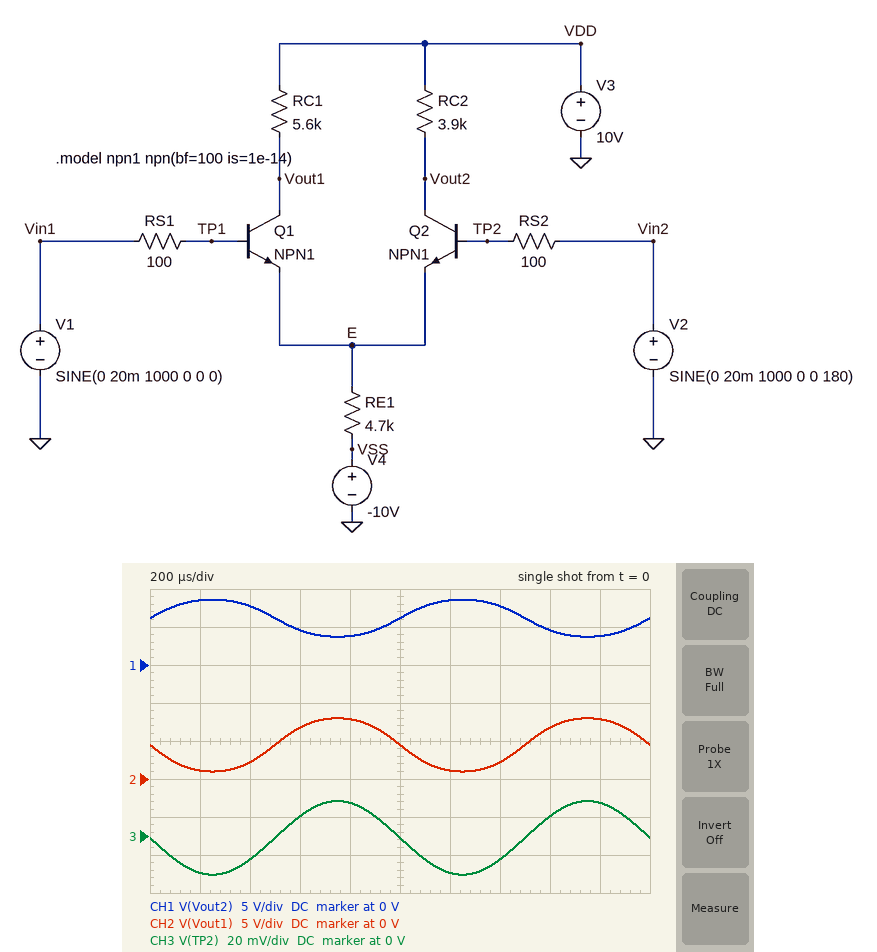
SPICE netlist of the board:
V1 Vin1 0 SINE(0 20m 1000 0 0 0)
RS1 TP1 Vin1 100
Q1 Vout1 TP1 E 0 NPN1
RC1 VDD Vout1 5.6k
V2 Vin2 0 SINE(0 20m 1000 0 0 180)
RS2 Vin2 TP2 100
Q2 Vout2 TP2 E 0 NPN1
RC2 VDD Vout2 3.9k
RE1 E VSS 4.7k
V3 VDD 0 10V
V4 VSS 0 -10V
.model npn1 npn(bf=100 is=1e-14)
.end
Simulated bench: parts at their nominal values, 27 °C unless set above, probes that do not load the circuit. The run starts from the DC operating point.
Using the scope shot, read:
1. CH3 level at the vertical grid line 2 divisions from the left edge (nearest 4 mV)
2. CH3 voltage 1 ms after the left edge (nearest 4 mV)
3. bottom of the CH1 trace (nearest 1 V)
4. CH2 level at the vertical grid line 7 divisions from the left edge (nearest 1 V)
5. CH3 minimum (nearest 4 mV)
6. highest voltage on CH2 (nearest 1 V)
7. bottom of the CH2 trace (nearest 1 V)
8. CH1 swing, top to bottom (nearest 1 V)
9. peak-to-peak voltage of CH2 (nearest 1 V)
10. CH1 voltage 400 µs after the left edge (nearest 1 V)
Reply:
-12 mV
0 V
4 V
2 V
-20 mV
8 V
1 V
5 V
7 V
8 V
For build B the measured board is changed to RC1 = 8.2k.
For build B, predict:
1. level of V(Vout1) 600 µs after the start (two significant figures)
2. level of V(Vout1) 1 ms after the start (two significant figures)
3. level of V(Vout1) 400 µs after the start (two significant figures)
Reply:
5.3 V
1.9 V
-560 mV
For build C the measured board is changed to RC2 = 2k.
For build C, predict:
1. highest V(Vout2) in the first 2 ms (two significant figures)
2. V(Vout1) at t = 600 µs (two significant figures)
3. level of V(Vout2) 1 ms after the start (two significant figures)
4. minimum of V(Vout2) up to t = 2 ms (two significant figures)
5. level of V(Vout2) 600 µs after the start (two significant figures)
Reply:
9.3 V
6.8 V
8.0 V
6.8 V
7.2 V
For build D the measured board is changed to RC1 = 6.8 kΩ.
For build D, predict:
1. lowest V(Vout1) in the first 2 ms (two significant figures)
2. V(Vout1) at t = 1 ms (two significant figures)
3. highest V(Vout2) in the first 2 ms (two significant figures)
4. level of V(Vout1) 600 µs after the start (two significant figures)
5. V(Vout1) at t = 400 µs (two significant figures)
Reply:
-540 mV
3.3 V
8.5 V
6.1 V
540 mV
